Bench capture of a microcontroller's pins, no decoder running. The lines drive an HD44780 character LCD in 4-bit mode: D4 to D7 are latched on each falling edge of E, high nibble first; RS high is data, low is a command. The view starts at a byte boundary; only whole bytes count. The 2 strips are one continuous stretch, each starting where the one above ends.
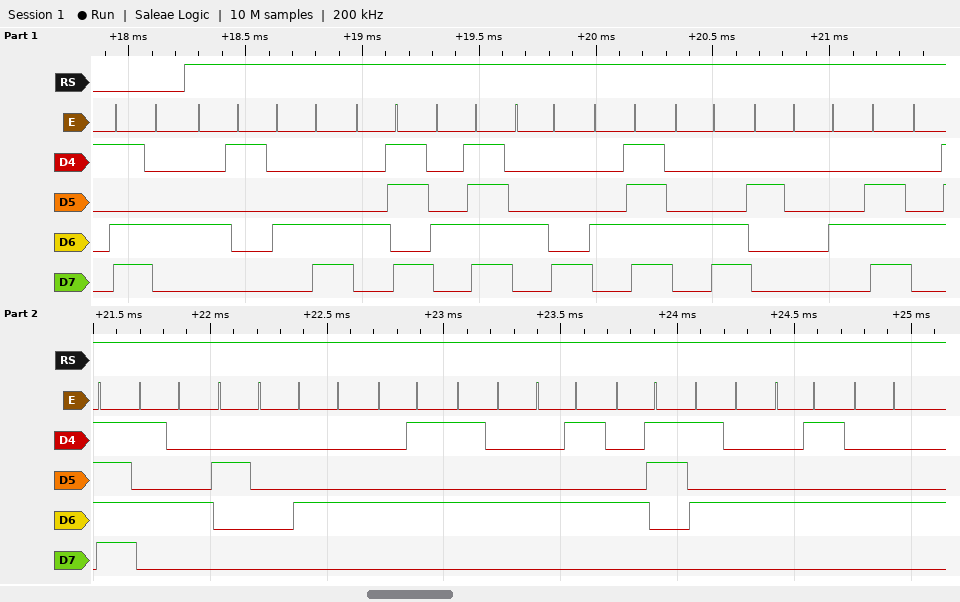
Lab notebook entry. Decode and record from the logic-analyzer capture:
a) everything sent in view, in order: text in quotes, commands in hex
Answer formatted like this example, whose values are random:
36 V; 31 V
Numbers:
0xD4 "ALKOHOL NOT DETECTED"
